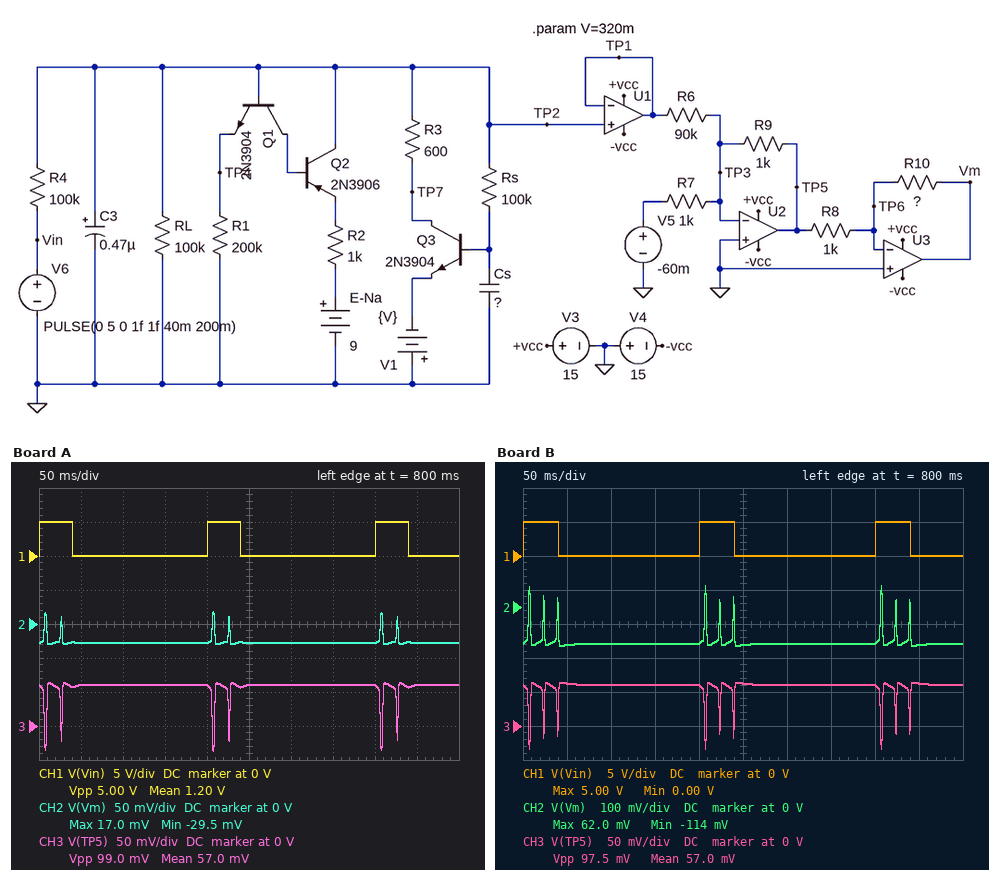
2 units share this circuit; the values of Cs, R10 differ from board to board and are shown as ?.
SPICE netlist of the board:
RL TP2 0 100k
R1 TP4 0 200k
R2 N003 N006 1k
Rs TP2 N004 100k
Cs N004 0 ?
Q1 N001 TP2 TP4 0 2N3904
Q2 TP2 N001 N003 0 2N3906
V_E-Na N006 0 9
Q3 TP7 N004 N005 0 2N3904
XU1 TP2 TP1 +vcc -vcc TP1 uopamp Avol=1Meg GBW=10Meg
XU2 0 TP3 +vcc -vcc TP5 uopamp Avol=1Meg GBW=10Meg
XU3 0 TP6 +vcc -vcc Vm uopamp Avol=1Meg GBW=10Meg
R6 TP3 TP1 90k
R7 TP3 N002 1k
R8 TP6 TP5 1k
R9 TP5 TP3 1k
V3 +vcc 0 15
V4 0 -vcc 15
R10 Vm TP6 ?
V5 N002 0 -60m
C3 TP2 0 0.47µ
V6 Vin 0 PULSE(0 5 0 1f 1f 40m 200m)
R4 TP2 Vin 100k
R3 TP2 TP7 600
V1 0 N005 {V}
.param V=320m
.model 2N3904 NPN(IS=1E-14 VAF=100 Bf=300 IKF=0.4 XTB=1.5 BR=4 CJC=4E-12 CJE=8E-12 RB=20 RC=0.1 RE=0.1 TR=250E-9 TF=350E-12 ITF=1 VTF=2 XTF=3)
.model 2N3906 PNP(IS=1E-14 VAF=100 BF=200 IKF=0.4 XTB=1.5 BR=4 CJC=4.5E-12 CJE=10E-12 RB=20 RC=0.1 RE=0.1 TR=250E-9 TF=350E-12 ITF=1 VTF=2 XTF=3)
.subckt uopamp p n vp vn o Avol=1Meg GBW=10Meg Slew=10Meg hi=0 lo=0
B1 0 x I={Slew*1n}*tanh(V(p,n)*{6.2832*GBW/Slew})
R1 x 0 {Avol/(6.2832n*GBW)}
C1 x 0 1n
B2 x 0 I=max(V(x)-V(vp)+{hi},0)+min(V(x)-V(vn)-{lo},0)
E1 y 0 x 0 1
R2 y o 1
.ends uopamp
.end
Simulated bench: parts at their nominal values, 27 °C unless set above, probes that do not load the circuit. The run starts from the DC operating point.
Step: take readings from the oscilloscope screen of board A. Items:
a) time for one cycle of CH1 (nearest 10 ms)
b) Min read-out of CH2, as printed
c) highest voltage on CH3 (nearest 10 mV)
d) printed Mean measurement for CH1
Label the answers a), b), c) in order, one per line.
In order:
a) 200 ms
b) -29.5 mV
c) 60 mV
d) 1.20 V
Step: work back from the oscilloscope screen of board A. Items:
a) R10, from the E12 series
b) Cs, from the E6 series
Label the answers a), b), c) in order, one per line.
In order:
a) 470 Ω
b) 680 nF
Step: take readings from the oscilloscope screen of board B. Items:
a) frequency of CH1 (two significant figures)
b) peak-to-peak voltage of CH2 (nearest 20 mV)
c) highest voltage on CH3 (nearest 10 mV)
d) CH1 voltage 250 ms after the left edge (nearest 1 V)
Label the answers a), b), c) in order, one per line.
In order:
a) 5.0 Hz
b) 180 mV
c) 60 mV
d) 0 V
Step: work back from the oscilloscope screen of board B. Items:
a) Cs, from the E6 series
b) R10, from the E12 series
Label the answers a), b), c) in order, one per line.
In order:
a) 470 nF
b) 1.8 kΩ
